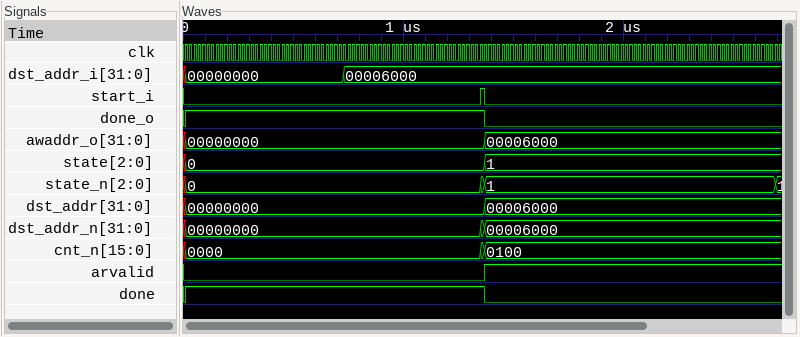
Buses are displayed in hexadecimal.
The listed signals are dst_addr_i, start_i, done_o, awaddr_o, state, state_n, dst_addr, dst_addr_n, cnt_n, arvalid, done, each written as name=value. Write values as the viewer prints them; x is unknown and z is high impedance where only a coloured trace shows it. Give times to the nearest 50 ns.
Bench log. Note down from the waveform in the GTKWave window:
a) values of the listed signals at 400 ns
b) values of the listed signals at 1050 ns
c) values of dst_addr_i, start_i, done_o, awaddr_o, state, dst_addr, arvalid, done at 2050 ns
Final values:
dst_addr_i=00000000, start_i=0, done_o=1, awaddr_o=00000000, state=0, state_n=0, dst_addr=00000000, dst_addr_n=00000000, cnt_n=0000, arvalid=0, done=1
dst_addr_i=00006000, start_i=0, done_o=1, awaddr_o=00000000, state=0, state_n=0, dst_addr=00000000, dst_addr_n=00000000, cnt_n=0000, arvalid=0, done=1
dst_addr_i=00006000, start_i=0, done_o=0, awaddr_o=00006000, state=1, dst_addr=00006000, arvalid=1, done=0
